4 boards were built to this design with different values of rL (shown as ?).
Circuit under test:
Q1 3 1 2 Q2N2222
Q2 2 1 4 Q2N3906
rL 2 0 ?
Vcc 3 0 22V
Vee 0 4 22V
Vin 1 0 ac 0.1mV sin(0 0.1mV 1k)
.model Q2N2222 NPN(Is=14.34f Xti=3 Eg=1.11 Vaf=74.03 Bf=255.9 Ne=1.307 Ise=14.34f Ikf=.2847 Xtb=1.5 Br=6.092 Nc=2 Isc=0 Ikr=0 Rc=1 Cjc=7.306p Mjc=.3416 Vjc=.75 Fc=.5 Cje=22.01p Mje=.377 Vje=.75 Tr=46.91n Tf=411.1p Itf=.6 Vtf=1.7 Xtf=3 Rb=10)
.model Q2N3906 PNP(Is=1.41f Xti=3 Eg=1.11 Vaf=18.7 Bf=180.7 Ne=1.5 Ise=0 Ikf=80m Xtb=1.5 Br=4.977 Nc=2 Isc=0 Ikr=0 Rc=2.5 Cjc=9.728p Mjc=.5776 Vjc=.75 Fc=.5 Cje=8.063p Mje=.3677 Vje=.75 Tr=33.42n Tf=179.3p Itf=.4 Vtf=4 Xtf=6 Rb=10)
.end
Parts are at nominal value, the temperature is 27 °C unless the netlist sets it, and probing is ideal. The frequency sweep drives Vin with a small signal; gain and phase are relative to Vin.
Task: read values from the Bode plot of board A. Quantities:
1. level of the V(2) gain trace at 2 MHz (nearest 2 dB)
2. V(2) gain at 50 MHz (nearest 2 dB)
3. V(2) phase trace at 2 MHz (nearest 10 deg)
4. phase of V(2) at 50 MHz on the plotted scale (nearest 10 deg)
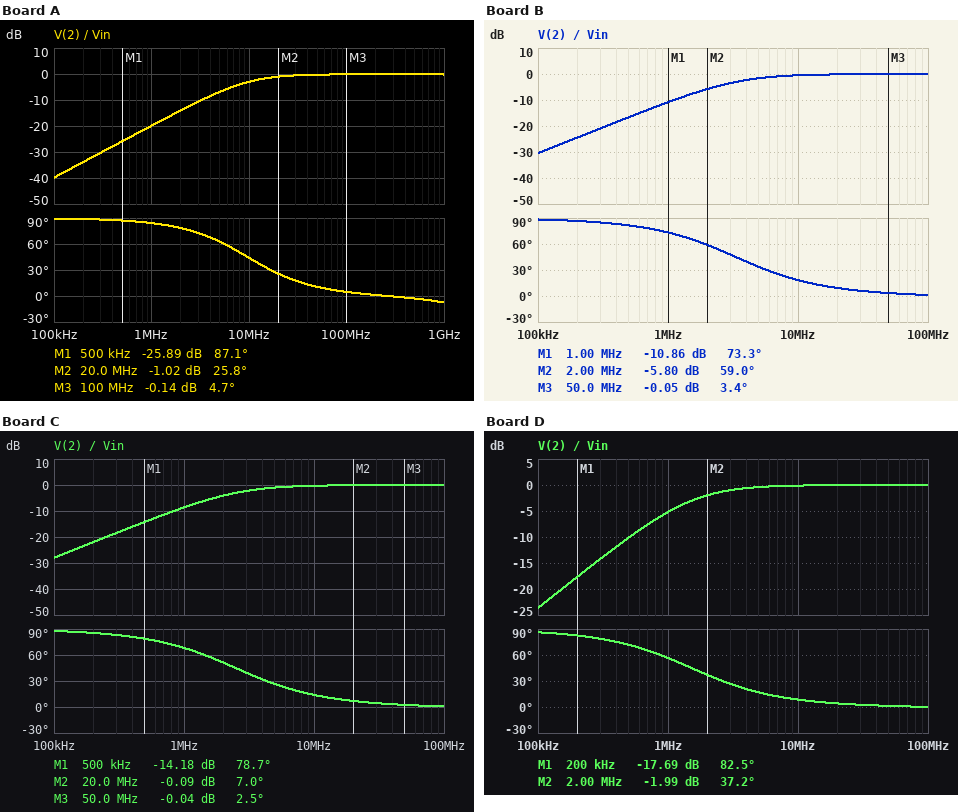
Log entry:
-14 dB
0 dB
80 deg
10 deg
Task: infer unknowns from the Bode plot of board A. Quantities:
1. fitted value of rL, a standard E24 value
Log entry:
510 Ω
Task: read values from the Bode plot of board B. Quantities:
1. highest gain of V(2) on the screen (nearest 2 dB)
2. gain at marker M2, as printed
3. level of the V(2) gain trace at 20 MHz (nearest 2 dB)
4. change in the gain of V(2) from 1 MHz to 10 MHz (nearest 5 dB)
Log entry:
0 dB
-5.80 dB
0 dB
10 dB
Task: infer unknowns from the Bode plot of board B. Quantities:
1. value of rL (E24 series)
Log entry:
1.5 kΩ
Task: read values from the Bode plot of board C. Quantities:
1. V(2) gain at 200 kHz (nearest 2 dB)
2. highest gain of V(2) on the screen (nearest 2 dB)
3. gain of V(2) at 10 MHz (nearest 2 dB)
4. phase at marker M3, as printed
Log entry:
-22 dB
0 dB
0 dB
2.5 deg
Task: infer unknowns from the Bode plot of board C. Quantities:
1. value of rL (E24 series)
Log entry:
2 kΩ
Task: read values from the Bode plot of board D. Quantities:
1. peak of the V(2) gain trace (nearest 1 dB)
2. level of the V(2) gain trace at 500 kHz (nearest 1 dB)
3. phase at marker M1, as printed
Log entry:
0 dB
-10 dB
82.5 deg
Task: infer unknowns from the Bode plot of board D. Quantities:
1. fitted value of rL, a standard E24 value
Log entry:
3.3 kΩ
